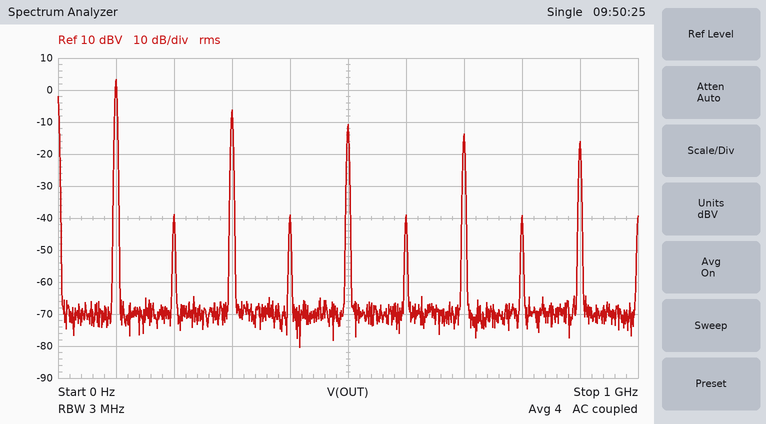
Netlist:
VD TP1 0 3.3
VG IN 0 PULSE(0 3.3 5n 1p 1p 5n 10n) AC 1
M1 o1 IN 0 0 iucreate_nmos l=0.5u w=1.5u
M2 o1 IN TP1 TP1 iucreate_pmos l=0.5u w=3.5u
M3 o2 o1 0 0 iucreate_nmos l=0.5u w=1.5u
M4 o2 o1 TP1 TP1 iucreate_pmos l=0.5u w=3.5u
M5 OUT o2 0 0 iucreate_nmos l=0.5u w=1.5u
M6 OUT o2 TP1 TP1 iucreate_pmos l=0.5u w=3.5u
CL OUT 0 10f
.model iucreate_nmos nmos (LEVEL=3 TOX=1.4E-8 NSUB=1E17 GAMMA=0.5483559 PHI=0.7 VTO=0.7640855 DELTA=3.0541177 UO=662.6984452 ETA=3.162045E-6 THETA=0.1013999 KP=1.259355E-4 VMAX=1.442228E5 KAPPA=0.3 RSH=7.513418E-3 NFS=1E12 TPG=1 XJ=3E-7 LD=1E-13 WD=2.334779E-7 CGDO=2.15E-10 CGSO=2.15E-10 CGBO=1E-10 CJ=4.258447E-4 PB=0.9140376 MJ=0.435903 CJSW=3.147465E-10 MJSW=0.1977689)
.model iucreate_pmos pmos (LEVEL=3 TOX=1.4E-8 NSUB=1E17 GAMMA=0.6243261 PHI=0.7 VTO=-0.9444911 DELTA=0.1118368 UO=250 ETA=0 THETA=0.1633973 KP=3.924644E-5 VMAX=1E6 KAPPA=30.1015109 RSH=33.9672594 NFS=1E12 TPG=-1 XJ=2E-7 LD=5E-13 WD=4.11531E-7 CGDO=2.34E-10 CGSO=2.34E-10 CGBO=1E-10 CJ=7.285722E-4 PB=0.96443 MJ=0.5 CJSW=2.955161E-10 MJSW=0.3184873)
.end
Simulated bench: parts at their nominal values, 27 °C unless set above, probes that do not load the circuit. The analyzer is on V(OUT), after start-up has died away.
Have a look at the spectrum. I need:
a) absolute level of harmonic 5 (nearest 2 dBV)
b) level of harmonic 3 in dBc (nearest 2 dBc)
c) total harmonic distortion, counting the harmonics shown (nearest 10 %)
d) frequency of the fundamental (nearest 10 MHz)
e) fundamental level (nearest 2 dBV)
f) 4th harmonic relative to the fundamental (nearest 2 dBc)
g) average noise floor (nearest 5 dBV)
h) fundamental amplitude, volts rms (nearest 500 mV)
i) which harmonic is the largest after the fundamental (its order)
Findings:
-10 dBV
-10 dBc
40 %
100 MHz
4 dBV
-42 dBc
-70 dBV
1.5 V
3
